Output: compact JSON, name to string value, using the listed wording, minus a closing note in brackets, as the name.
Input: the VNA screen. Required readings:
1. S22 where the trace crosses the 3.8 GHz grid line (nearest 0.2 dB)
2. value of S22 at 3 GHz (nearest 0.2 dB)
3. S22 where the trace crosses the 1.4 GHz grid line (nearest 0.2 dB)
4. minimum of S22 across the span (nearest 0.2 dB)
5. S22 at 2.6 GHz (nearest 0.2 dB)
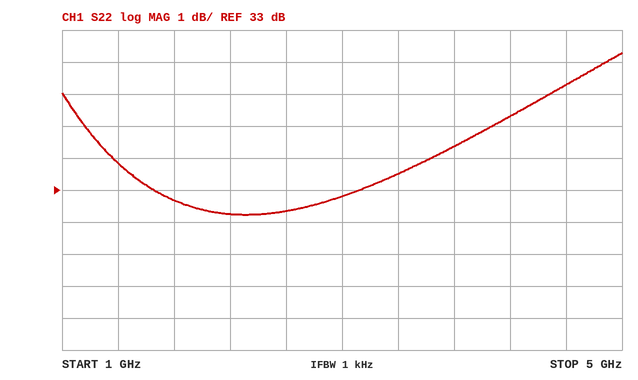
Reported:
{"S22 where the trace crosses the 3.8 GHz grid line": "34.4 dB", "value of S22 at 3 GHz": "32.8 dB", "S22 where the trace crosses the 1.4 GHz grid line": "33.8 dB", "minimum of S22 across the span": "32.2 dB", "S22 at 2.6 GHz": "32.4 dB"}
